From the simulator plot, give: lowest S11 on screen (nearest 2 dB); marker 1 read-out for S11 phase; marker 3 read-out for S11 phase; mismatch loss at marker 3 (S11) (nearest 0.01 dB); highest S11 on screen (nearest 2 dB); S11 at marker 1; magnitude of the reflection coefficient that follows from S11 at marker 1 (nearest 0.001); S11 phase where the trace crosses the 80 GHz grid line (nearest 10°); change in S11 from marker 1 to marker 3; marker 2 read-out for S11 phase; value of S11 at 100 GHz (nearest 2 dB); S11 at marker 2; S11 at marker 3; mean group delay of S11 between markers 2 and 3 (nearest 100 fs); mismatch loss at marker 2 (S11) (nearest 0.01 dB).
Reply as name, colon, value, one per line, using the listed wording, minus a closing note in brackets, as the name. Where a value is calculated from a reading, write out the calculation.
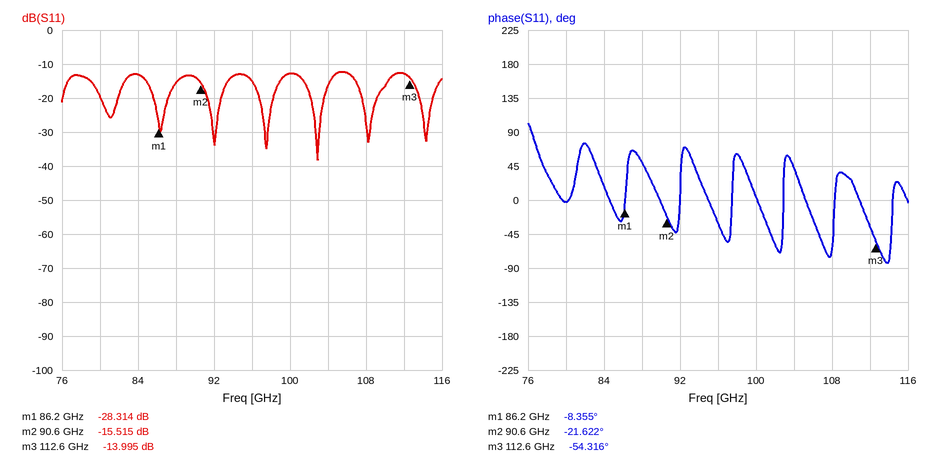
lowest S11 on screen: -38 dB
marker 1 read-out for S11 phase: -8.355°
marker 3 read-out for S11 phase: -54.316°
mismatch loss at marker 3 (S11): −10 log10(1 − 10^(-13.995/10)) ≈ 0.18 dB
highest S11 on screen: -12 dB
S11 at marker 1: -28.314 dB
magnitude of the reflection coefficient that follows from S11 at marker 1: 10^(-28.314/20) ≈ 0.038
S11 phase where the trace crosses the 80 GHz grid line: 0°
change in S11 from marker 1 to marker 3: -13.995 − (-28.314) = 14.319 dB
marker 2 read-out for S11 phase: -21.622°
value of S11 at 100 GHz: -12 dB
S11 at marker 2: -15.515 dB
S11 at marker 3: -13.995 dB
mean group delay of S11 between markers 2 and 3: −(-54.316° − (-21.622°))/(360° × 22 GHz) ≈ 4.1 ps
mismatch loss at marker 2 (S11): −10 log10(1 − 10^(-15.515/10)) ≈ 0.12 dB
